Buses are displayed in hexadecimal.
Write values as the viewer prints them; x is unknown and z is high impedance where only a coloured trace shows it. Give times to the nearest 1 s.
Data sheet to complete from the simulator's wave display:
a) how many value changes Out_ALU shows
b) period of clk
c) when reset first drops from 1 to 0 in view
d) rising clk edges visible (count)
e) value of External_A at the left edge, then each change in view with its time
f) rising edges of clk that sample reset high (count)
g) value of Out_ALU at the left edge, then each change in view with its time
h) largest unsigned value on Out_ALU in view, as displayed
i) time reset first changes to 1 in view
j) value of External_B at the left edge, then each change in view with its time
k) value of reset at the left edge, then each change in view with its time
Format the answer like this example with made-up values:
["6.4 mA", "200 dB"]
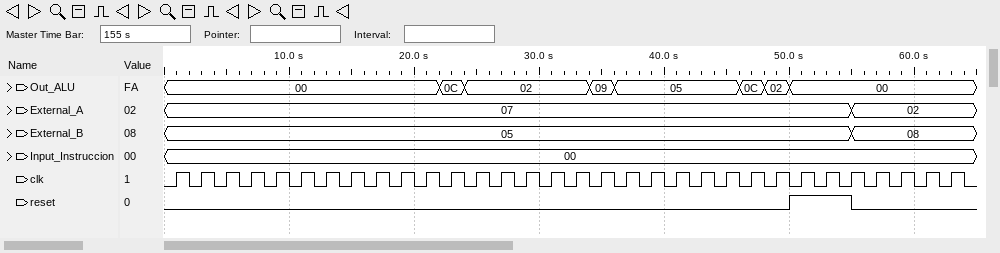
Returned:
["7", "2 s", "55 s", "32", "07, 02 at 55 s", "3", "00, 0C at 22 s, 02 at 24 s, 09 at 34 s, 05 at 36 s, 0C at 46 s, 02 at 48 s, 00 at 50 s", "0C", "50 s", "05, 08 at 55 s", "0, 1 at 50 s, 0 at 55 s"]
